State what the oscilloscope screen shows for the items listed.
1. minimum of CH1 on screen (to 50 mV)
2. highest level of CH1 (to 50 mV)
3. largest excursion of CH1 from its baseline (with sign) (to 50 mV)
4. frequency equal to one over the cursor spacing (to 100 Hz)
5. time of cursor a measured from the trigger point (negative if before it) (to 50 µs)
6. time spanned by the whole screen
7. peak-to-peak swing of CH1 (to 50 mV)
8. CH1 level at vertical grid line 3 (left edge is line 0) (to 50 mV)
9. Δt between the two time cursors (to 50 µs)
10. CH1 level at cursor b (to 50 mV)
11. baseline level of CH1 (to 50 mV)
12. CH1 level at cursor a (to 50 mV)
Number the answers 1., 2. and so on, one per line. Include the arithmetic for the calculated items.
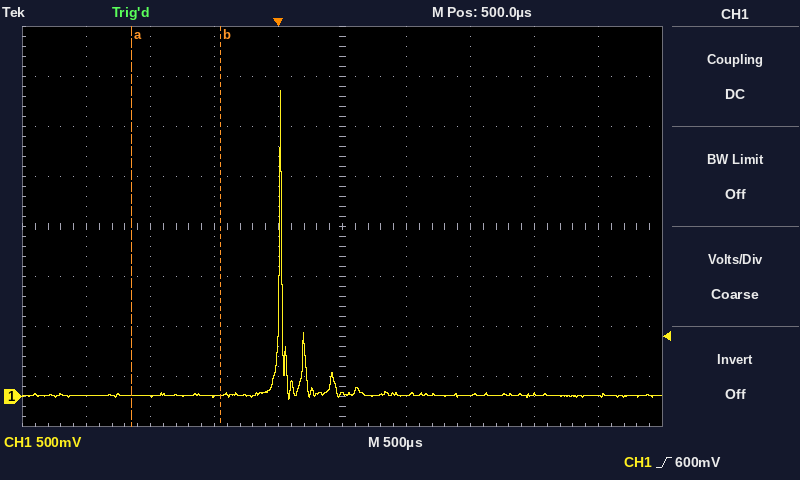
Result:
1. -50 mV
2. 3.05 V
3. 3.05 V − (0 mV) = +3.05 V
4. 1 / 700 µs ≈ 1.4 kHz
5. -1.15 ms
6. 5 ms
7. 3.05 V − (-50 mV) = 3.10 V
8. 0 mV
9. 700 µs
10. 0 mV
11. 0 mV
12. 0 mV
